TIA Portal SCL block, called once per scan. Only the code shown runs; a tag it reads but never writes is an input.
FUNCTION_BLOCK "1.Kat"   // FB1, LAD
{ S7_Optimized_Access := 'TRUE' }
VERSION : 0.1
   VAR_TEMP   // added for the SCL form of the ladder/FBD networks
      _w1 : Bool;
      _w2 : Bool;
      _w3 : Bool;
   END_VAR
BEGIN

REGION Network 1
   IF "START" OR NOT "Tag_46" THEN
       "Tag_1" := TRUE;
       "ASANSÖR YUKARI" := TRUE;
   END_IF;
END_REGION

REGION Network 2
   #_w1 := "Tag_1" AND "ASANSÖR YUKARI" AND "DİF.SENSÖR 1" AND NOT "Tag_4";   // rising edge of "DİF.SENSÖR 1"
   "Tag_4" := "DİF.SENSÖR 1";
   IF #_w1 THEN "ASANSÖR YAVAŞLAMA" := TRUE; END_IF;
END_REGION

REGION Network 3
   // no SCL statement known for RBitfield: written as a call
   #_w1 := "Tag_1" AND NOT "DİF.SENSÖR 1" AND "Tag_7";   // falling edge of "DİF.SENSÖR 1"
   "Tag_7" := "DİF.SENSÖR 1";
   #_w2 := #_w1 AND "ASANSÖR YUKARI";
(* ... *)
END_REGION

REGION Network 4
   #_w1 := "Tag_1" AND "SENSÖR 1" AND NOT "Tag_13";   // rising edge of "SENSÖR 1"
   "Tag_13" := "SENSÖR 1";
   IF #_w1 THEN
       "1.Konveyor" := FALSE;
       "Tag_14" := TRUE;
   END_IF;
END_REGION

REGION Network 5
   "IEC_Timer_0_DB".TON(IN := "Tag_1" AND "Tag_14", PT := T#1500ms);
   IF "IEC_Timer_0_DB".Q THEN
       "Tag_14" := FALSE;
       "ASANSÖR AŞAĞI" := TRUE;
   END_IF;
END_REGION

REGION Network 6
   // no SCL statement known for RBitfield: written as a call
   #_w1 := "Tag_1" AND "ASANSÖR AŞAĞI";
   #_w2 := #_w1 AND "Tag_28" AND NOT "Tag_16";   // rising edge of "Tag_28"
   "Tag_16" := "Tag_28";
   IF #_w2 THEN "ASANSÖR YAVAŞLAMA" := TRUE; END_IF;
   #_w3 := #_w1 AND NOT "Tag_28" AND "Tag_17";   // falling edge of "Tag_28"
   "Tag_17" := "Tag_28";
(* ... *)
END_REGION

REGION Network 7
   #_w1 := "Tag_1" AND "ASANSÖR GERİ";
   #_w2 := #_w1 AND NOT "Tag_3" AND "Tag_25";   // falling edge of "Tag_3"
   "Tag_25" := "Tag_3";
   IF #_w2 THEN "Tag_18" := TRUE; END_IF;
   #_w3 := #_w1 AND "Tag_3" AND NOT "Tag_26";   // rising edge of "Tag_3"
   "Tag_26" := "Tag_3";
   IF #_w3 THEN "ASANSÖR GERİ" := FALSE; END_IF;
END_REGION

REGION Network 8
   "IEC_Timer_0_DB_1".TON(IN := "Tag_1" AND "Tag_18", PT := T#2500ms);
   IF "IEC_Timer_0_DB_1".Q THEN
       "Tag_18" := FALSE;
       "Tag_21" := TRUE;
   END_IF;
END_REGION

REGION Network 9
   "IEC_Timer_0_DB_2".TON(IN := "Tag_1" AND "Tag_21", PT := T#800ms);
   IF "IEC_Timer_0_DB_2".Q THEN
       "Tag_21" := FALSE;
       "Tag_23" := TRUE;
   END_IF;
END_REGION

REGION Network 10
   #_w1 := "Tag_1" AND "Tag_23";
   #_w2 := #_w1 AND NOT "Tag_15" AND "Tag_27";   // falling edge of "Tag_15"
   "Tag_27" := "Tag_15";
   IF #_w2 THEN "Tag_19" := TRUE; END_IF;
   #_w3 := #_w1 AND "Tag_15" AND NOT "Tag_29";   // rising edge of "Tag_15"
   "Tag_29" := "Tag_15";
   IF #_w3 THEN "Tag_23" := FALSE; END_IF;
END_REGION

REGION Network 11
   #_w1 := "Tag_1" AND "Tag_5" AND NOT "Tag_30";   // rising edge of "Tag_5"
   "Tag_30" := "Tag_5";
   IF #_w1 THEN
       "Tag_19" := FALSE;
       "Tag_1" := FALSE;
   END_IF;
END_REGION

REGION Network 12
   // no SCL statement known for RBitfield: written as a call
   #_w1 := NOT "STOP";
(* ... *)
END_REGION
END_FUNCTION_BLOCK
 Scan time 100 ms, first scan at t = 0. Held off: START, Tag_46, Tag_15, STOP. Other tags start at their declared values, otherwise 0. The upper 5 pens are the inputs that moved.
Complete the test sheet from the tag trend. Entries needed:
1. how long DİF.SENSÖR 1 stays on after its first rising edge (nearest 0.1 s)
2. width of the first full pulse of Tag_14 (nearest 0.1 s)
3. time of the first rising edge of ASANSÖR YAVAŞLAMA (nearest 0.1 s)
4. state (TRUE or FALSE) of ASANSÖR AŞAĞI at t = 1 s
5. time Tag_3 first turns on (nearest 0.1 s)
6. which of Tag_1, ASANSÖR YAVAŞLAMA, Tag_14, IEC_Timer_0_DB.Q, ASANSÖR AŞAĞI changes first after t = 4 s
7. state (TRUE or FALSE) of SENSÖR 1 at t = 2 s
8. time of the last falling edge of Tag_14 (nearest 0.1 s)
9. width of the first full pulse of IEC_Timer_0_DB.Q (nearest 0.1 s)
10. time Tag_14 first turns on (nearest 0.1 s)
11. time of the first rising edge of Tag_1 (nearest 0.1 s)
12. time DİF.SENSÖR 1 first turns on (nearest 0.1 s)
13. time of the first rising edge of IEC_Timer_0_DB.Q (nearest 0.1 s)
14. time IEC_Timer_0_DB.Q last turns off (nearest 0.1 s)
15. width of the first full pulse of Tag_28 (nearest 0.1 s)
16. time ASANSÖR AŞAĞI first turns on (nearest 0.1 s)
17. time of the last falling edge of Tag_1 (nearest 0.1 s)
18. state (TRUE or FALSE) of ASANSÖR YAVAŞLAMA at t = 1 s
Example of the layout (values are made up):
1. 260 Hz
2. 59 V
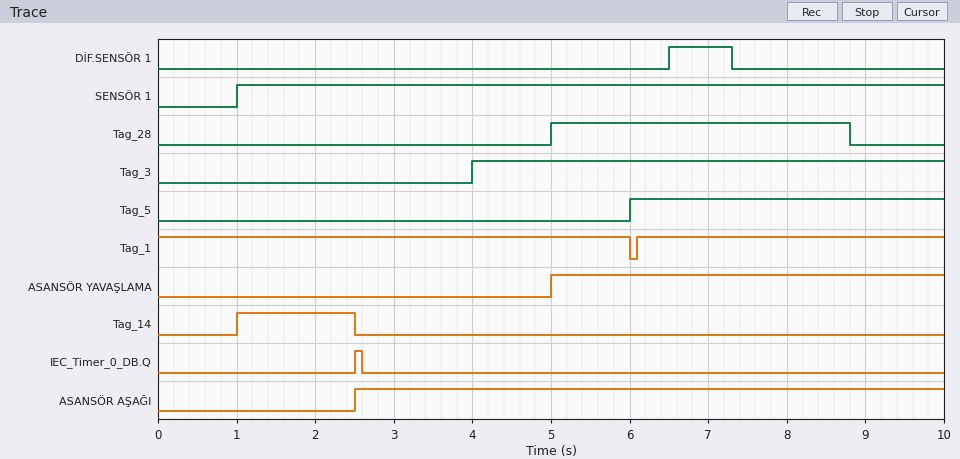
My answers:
1. 0.8 s
2. 1.5 s
3. 5.0 s
4. FALSE
5. 4.0 s
6. ASANSÖR YAVAŞLAMA
7. TRUE
8. 2.5 s
9. 0.1 s
10. 1.0 s
11. 6.1 s
12. 6.5 s
13. 2.5 s
14. 2.6 s
15. 3.8 s
16. 2.5 s
17. 6.0 s
18. FALSE
